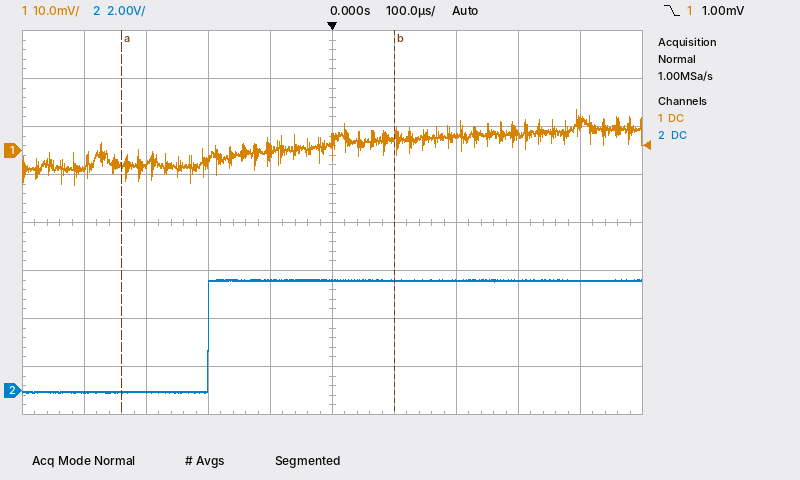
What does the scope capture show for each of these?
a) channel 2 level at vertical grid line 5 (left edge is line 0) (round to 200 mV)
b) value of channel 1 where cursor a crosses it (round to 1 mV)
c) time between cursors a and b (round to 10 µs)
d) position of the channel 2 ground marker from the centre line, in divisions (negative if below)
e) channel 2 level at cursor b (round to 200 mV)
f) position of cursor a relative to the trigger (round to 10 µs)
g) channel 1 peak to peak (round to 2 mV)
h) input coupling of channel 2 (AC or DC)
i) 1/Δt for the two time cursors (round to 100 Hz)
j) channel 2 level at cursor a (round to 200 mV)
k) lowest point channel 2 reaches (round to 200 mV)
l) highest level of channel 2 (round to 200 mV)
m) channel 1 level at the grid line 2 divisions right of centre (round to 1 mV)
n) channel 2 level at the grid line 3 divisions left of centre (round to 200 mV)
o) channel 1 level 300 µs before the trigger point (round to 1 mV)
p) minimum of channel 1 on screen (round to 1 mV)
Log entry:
4.6 V
-3 mV
440 µs
-3.5 div
4.6 V
-340 µs
16 mV
DC
2.3 kHz
0.0 V
0.0 V
4.6 V
3 mV
0.0 V
-3 mV
-7 mV
